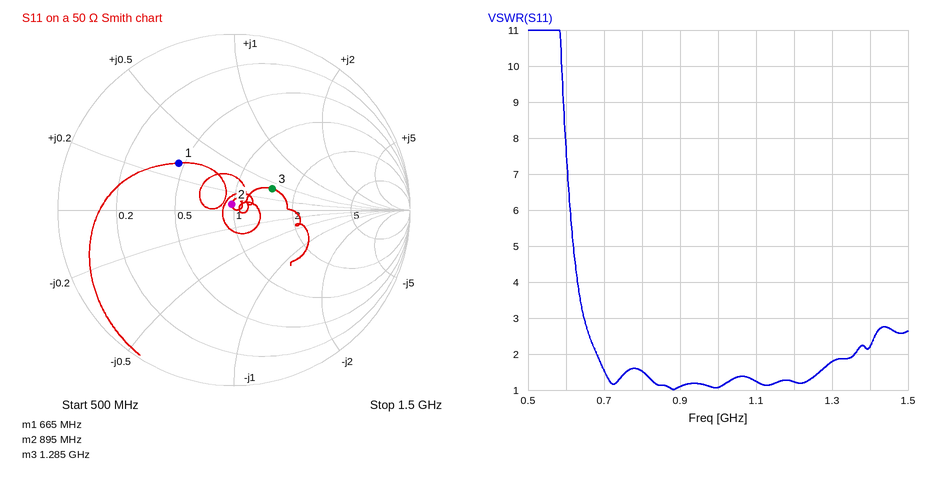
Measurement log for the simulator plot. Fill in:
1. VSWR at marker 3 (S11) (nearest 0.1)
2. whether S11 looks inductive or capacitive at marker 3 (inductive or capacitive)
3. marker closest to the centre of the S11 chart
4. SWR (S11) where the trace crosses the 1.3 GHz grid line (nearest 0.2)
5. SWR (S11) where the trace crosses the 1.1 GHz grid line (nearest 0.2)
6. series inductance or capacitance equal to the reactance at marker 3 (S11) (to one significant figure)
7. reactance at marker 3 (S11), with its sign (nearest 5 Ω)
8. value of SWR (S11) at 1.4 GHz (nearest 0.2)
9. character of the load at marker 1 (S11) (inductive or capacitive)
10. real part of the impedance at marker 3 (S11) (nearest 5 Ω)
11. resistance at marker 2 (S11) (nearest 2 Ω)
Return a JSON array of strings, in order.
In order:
["1.7", "inductive", "marker 2", "1.8", "1.2", "2 nH", "+20 Ω", "2.2", "inductive", "75 Ω", "48 Ω"]
